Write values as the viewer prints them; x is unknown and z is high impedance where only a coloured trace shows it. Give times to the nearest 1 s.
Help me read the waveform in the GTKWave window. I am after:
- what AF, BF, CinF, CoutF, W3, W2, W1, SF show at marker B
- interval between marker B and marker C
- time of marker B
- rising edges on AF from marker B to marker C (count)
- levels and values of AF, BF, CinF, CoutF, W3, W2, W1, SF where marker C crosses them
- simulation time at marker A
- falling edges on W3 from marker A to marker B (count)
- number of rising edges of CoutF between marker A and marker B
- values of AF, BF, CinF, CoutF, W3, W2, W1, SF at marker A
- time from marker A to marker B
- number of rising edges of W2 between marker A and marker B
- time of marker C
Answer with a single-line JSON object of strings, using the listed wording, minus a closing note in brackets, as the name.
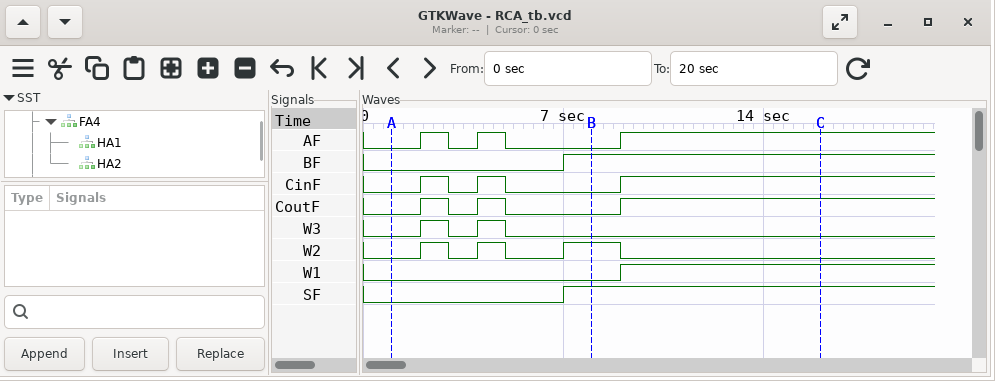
{"what AF, BF, CinF, CoutF, W3, W2, W1, SF show at marker B": "AF=0, BF=1, CinF=0, CoutF=0, W3=0, W2=1, W1=0, SF=1", "interval between marker B and marker C": "8 s", "time of marker B": "8 s", "rising edges on AF from marker B to marker C": "1", "levels and values of AF, BF, CinF, CoutF, W3, W2, W1, SF where marker C crosses them": "AF=1, BF=1, CinF=1, CoutF=1, W3=0, W2=0, W1=1, SF=1", "simulation time at marker A": "1 s", "falling edges on W3 from marker A to marker B": "2", "number of rising edges of CoutF between marker A and marker B": "2", "values of AF, BF, CinF, CoutF, W3, W2, W1, SF at marker A": "AF=0, BF=0, CinF=0, CoutF=0, W3=0, W2=0, W1=0, SF=0", "time from marker A to marker B": "7 s", "number of rising edges of W2 between marker A and marker B": "3", "time of marker C": "16 s"}
